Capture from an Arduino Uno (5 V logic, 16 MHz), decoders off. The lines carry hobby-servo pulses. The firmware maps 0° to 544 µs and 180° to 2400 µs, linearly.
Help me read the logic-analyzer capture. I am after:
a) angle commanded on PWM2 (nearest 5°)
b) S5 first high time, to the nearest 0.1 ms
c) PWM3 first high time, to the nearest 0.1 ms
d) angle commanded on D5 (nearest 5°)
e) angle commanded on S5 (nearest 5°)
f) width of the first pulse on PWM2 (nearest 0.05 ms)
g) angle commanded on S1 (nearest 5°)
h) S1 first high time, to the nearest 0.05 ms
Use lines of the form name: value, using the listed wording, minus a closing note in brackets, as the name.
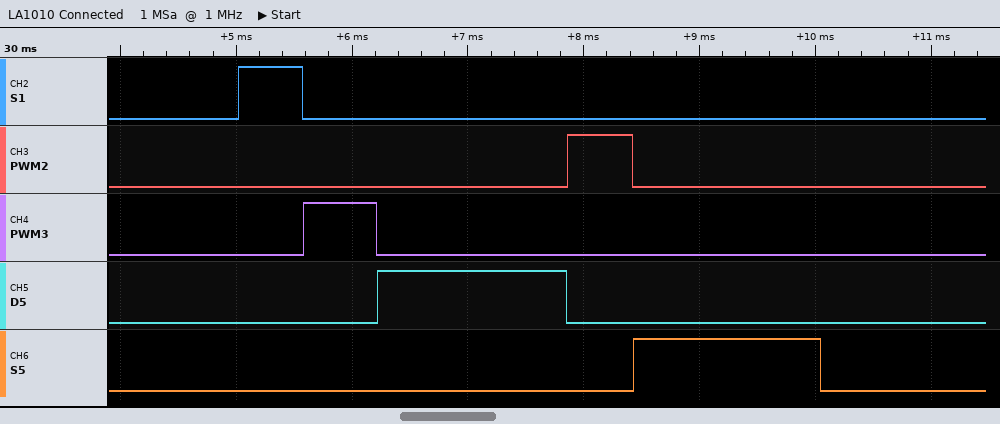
angle commanded on PWM2: 0°
S5 first high time, to the nearest 0.1 ms: 1.6 ms
PWM3 first high time, to the nearest 0.1 ms: 0.6 ms
angle commanded on D5: 105°
angle commanded on S5: 105°
width of the first pulse on PWM2: 0.55 ms
angle commanded on S1: 0°
S1 first high time, to the nearest 0.05 ms: 0.55 ms
